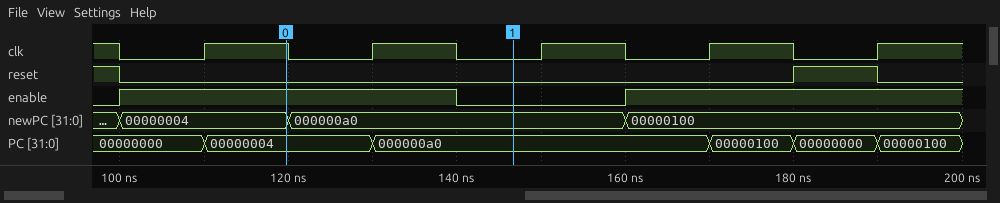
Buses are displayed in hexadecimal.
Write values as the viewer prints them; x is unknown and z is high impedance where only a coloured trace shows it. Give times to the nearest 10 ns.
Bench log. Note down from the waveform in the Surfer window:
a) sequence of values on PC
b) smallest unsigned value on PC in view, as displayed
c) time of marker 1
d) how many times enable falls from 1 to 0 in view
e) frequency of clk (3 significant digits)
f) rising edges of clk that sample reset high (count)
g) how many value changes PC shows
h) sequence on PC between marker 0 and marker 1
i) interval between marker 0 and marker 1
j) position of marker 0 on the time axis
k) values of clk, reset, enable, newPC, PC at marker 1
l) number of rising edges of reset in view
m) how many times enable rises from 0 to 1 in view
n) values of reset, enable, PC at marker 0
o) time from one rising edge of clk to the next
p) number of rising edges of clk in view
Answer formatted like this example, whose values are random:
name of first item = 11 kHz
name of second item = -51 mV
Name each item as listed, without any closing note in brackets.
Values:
sequence of values on PC = 00000000, 00000004, 000000a0, 00000100, 00000000, 00000100
smallest unsigned value on PC in view, as displayed = 00000000
time of marker 1 = 150 ns
how many times enable falls from 1 to 0 in view = 1
frequency of clk = 50.0 MHz
rising edges of clk that sample reset high = 1
how many value changes PC shows = 5
sequence on PC between marker 0 and marker 1 = 00000004, 000000a0
interval between marker 0 and marker 1 = 30 ns
position of marker 0 on the time axis = 120 ns
values of clk, reset, enable, newPC, PC at marker 1 = clk=0, reset=0, enable=0, newPC=000000a0, PC=000000a0
number of rising edges of reset in view = 1
how many times enable rises from 0 to 1 in view = 2
values of reset, enable, PC at marker 0 = reset=0, enable=1, PC=00000004
time from one rising edge of clk to the next = 20 ns
number of rising edges of clk in view = 5
